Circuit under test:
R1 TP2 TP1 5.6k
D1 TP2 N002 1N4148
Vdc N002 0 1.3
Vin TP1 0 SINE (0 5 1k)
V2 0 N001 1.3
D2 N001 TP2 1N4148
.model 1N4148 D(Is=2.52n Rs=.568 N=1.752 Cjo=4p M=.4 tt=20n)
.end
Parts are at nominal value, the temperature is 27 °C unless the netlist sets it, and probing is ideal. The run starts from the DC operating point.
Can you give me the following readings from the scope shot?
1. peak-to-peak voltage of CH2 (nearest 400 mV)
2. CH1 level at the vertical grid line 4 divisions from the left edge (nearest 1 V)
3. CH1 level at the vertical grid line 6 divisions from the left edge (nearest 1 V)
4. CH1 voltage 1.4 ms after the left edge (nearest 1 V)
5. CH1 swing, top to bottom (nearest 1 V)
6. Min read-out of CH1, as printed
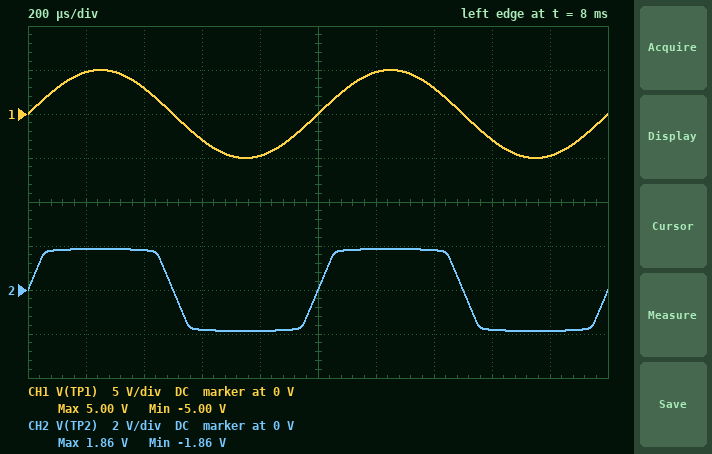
3.6 V
-5 V
5 V
3 V
10 V
-5.00 V
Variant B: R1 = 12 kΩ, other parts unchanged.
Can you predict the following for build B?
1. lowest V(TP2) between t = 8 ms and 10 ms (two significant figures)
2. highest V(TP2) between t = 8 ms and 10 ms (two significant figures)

-1.8 V
1.8 V
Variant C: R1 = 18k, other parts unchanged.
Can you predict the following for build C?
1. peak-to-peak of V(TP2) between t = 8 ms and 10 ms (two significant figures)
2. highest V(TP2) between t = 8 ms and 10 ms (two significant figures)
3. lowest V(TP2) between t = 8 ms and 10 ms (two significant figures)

3.6 V
1.8 V
-1.8 V
